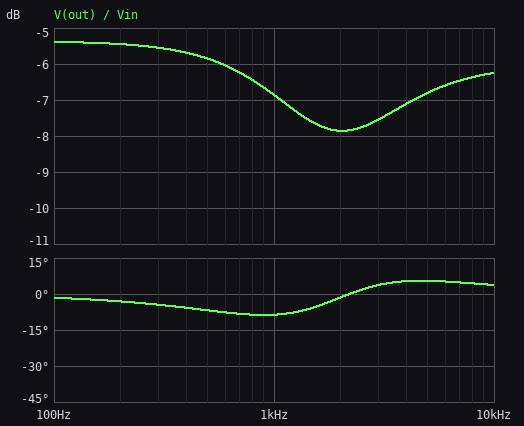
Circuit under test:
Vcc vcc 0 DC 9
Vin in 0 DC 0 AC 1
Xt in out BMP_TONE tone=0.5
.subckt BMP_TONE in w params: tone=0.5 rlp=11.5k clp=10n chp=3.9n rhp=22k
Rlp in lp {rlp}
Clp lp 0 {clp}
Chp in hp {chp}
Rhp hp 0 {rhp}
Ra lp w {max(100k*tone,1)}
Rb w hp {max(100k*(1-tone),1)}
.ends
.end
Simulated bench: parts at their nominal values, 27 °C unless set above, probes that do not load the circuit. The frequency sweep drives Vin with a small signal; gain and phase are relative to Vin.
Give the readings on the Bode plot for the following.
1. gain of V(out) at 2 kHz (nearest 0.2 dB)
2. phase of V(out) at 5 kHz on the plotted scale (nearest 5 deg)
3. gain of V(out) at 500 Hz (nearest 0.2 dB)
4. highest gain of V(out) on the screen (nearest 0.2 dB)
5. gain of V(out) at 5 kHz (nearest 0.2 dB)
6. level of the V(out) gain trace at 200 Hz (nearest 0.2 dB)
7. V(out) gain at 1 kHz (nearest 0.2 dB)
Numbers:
-7.8 dB
5 deg
-5.8 dB
-5.4 dB
-6.8 dB
-5.4 dB
-6.8 dB
